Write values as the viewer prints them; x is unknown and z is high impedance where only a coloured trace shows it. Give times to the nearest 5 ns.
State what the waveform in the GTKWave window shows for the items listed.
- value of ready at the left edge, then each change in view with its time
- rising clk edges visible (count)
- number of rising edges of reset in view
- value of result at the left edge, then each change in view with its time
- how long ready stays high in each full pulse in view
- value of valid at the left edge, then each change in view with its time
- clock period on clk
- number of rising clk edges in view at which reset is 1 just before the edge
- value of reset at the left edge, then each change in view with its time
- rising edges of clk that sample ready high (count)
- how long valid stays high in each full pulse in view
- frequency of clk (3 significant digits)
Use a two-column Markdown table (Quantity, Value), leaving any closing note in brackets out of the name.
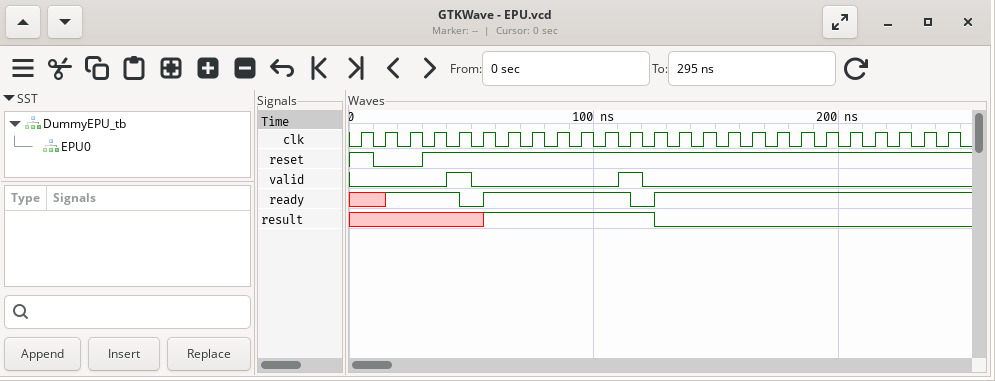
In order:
| Quantity | Value |
|---|---|
| value of ready at the left edge, then each change in view with its time | x, 1 at 15 ns, 0 at 45 ns, 1 at 55 ns, 0 at 115 ns, 1 at 125 ns |
| rising clk edges visible | 25 |
| number of rising edges of reset in view | 1 |
| value of result at the left edge, then each change in view with its time | x, 1 at 55 ns, 0 at 125 ns |
| how long ready stays high in each full pulse in view | 60 ns |
| value of valid at the left edge, then each change in view with its time | 0, 1 at 40 ns, 0 at 50 ns, 1 at 110 ns, 0 at 120 ns |
| clock period on clk | 10 ns |
| number of rising clk edges in view at which reset is 1 just before the edge | 23 |
| value of reset at the left edge, then each change in view with its time | 1, 0 at 10 ns, 1 at 30 ns |
| rising edges of clk that sample ready high | 21 |
| how long valid stays high in each full pulse in view | 10 ns, 10 ns |
| frequency of clk | 100 MHz |
